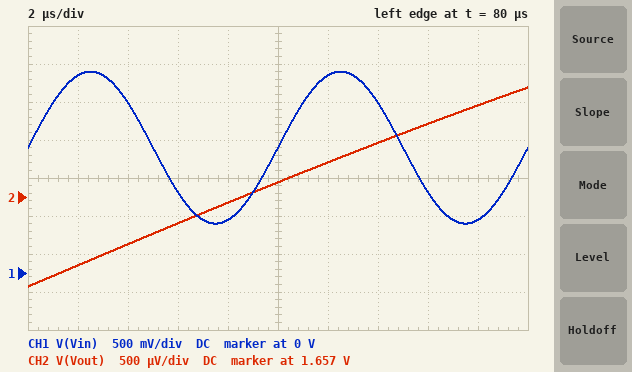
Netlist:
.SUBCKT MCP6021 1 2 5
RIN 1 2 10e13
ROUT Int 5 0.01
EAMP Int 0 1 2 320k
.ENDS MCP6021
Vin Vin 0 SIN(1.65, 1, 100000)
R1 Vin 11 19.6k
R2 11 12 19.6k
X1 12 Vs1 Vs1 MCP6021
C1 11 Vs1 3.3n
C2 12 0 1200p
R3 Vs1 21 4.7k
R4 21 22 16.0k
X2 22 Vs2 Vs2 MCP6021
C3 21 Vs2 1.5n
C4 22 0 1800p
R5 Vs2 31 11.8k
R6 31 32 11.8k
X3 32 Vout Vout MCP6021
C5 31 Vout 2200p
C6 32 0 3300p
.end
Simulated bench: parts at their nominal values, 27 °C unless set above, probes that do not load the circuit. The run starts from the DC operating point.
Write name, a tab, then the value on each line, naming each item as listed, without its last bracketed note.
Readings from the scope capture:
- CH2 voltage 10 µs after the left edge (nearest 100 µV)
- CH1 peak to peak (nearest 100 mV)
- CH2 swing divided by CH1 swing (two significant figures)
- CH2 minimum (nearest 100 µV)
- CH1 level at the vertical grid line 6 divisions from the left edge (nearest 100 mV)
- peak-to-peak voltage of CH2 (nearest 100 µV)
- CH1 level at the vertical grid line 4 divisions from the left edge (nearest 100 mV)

CH2 voltage 10 µs after the left edge	1.6567 V
CH1 peak to peak	2.0 V
CH2 swing divided by CH1 swing	0.0013
CH2 minimum	1.6553 V
CH1 level at the vertical grid line 6 divisions from the left edge	2.6 V
peak-to-peak voltage of CH2	2.6 mV
CH1 level at the vertical grid line 4 divisions from the left edge	700 mV
